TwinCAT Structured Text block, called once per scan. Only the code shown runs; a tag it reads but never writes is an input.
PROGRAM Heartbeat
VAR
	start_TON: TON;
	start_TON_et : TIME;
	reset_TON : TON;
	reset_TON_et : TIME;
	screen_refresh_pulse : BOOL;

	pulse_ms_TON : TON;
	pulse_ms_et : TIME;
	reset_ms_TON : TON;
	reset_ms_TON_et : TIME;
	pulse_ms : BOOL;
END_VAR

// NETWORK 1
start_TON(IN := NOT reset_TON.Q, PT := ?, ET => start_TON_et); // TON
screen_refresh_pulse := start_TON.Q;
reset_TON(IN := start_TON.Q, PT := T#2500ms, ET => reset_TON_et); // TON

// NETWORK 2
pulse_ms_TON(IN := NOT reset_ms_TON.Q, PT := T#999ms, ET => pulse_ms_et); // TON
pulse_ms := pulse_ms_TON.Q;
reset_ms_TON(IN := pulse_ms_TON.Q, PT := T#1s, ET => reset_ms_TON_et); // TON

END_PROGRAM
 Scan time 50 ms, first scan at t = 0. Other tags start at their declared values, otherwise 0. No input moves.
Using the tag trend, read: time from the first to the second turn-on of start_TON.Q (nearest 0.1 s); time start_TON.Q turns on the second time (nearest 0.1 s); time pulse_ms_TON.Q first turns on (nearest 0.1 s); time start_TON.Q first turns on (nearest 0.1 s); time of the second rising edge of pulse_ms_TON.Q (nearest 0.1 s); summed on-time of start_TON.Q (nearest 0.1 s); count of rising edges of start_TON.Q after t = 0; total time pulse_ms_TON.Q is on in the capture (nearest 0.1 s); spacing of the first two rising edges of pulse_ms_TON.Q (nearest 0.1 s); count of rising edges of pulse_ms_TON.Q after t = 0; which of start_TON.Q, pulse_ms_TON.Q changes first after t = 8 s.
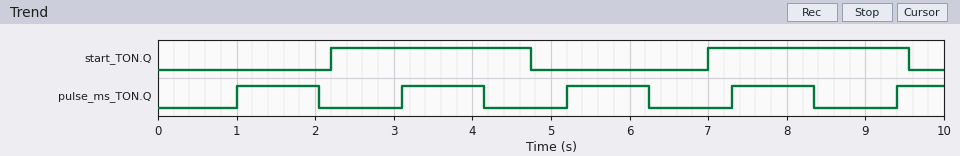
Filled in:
4.8 s
7.0 s
1.0 s
2.2 s
3.1 s
5.1 s
2
4.8 s
2.1 s
5
pulse_ms_TON.Q
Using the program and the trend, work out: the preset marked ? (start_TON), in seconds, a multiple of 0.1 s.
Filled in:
2.2 s
